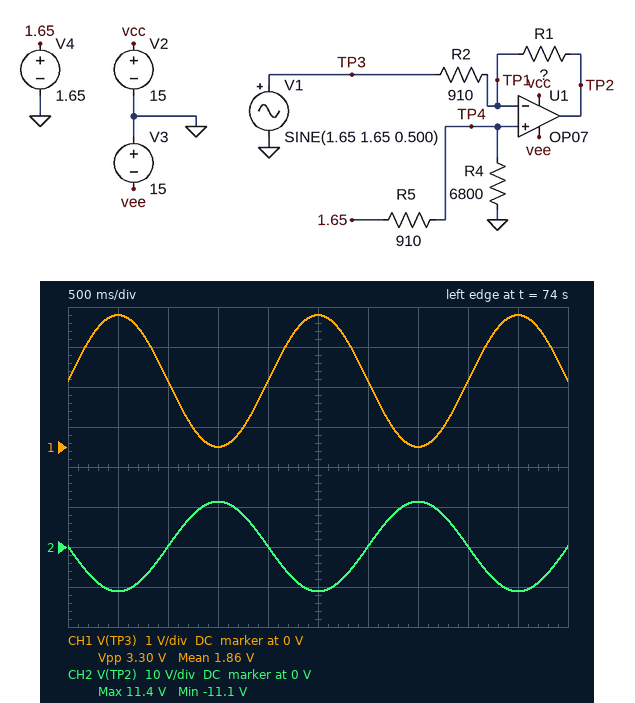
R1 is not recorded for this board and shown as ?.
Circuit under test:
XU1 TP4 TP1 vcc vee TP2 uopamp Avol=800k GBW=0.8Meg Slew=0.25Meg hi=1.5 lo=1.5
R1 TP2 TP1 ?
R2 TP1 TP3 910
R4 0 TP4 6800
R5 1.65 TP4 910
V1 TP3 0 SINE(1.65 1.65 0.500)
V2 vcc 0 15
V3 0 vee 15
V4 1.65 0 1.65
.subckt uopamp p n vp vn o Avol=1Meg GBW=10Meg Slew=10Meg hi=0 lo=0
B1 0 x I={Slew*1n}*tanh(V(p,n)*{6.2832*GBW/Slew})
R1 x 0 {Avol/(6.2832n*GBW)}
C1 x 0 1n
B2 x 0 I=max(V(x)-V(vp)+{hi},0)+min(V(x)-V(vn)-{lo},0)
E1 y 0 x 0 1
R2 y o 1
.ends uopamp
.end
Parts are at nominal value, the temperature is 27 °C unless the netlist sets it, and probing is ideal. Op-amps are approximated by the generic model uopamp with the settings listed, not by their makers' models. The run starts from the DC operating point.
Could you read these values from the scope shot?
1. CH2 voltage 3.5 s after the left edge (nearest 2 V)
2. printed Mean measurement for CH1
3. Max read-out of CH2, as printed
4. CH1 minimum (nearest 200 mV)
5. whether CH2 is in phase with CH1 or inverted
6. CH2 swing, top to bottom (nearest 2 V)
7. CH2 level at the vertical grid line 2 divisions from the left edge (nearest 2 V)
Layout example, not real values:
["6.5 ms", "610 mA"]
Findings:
["12 V", "1.86 V", "11.4 V", "0 V", "inverted", "22 V", "0 V"]
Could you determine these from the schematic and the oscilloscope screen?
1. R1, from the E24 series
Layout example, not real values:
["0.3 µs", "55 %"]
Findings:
["6.2 kΩ"]
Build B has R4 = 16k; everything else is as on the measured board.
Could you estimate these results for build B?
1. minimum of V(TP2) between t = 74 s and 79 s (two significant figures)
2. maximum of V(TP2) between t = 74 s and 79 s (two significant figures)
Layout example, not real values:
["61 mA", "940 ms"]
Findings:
["-10 V", "12 V"]
